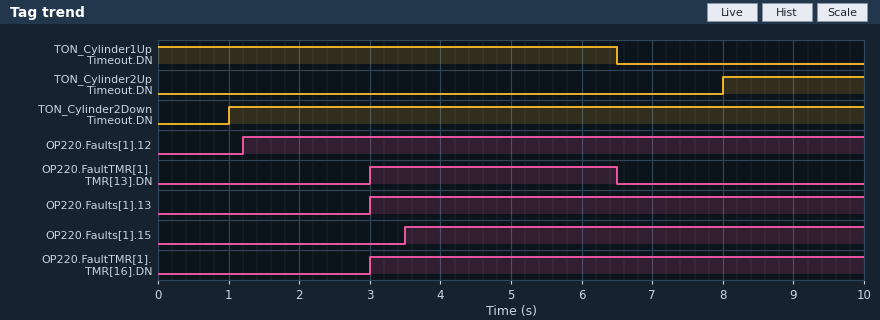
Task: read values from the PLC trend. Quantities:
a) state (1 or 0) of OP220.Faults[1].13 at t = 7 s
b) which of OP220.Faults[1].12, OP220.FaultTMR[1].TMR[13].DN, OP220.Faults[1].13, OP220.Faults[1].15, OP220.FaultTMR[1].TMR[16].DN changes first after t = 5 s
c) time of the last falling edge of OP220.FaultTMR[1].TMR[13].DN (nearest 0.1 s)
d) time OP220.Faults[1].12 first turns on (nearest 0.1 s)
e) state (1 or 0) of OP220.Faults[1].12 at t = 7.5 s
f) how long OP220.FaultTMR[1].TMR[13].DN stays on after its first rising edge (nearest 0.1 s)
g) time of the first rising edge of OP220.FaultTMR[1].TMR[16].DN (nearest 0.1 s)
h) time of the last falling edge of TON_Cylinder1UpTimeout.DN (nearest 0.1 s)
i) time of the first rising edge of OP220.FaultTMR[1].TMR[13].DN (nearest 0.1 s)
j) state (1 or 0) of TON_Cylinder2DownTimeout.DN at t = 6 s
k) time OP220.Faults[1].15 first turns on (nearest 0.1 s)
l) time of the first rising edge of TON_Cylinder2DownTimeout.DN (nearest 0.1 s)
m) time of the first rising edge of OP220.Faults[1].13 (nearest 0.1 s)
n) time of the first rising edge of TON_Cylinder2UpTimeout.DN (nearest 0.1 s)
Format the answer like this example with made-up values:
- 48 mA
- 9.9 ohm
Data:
- 1
- OP220.FaultTMR[1].TMR[13].DN
- 6.5 s
- 1.2 s
- 1
- 3.5 s
- 3.0 s
- 6.5 s
- 3.0 s
- 1
- 3.5 s
- 1.0 s
- 3.0 s
- 8.0 s
